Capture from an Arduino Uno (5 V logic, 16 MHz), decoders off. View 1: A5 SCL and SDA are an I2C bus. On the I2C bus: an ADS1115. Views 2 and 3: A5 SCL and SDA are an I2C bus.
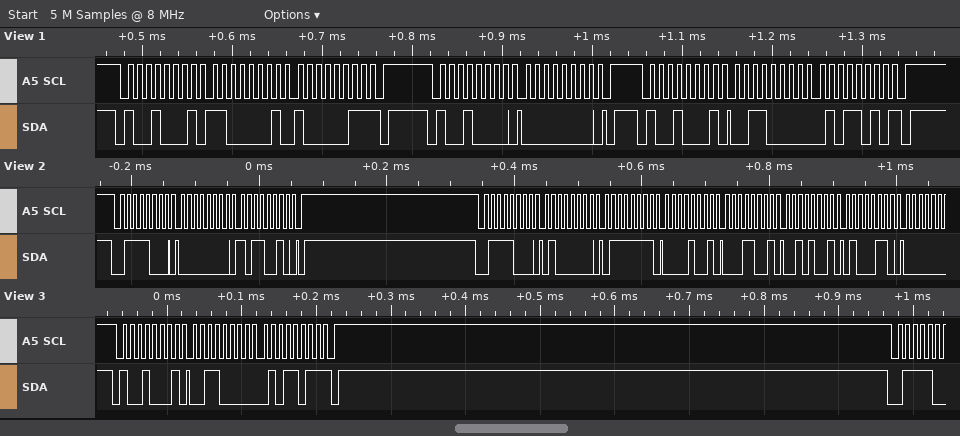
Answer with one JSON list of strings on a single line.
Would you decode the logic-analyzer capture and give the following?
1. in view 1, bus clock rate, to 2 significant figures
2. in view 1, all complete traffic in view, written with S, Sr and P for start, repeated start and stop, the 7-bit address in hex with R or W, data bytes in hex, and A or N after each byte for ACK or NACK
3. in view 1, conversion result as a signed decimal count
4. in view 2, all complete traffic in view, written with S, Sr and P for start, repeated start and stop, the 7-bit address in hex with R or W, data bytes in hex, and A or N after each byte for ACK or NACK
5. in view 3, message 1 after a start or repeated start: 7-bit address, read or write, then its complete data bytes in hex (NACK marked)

["100 kHz", "S 48R A C1 A 83 N P S 48W A 00 A P S 48R A 30 A 5A N P", "12378", "S 3CW A 00 A B2 A P S 3CW A 40 A 7F A 09 A 19 A 29 A 46 A", "0x48 read: 30 5B NACK"]
